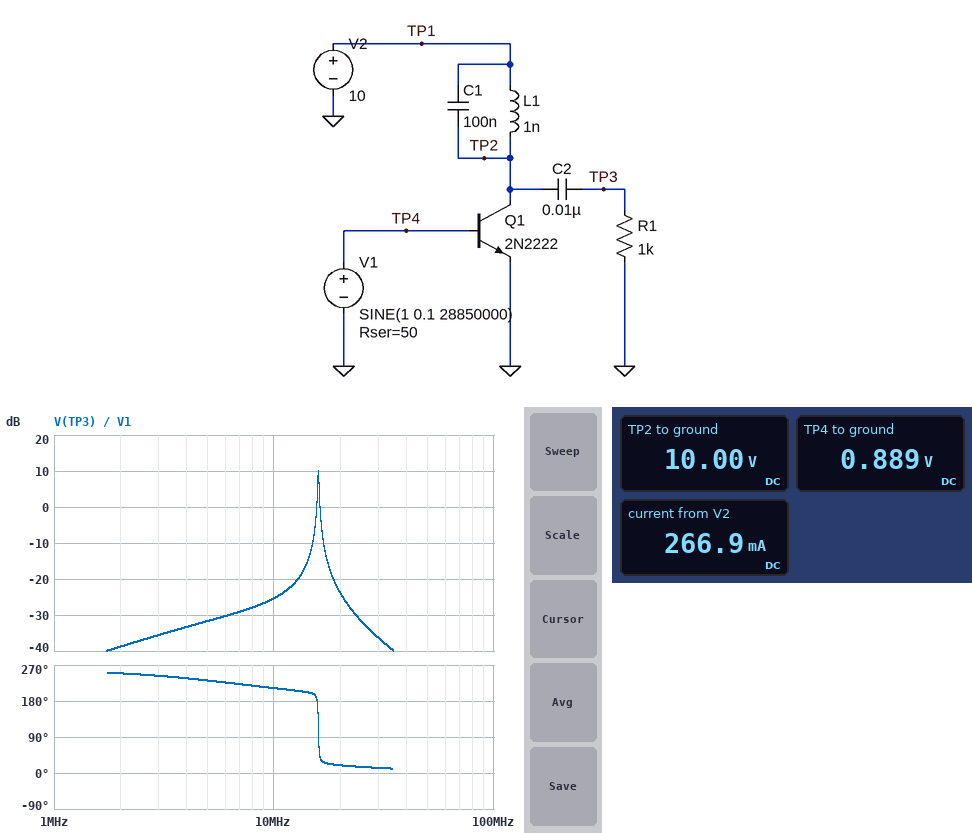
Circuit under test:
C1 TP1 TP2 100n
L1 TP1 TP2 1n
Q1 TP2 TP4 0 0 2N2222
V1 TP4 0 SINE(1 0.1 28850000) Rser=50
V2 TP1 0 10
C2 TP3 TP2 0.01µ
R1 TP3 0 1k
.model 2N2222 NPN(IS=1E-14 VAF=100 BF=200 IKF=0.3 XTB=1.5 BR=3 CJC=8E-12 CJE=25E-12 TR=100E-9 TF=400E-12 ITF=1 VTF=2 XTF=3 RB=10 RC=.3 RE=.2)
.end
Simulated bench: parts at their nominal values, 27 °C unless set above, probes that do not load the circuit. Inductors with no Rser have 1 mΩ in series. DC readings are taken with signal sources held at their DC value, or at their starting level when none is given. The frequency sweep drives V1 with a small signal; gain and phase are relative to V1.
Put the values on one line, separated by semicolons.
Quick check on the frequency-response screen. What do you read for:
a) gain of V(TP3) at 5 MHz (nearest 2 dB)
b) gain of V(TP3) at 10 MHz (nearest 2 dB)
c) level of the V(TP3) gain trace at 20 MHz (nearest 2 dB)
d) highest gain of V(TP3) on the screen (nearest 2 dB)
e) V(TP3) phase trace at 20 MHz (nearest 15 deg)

-32 dB; -26 dB; -24 dB; 10 dB; 15 deg
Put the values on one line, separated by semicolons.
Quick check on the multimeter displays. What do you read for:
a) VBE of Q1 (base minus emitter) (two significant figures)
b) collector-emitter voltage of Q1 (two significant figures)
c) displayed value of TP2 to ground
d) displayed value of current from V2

890 mV; 10 V; 10.00 V; 266.9 mA
